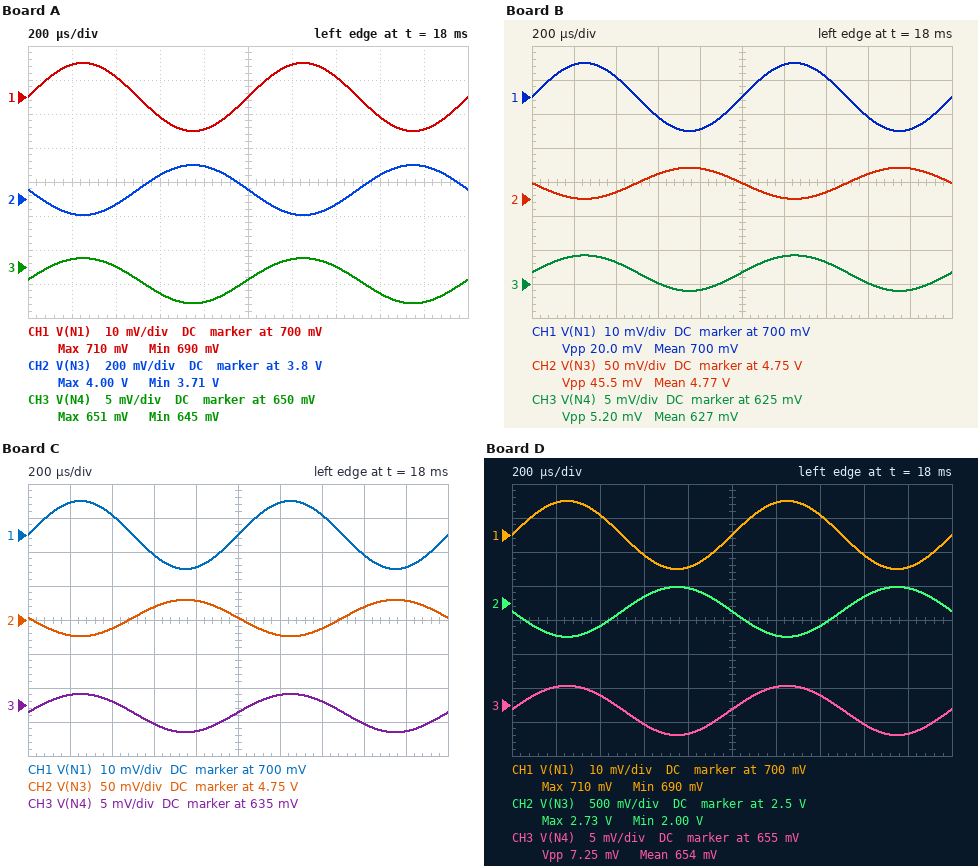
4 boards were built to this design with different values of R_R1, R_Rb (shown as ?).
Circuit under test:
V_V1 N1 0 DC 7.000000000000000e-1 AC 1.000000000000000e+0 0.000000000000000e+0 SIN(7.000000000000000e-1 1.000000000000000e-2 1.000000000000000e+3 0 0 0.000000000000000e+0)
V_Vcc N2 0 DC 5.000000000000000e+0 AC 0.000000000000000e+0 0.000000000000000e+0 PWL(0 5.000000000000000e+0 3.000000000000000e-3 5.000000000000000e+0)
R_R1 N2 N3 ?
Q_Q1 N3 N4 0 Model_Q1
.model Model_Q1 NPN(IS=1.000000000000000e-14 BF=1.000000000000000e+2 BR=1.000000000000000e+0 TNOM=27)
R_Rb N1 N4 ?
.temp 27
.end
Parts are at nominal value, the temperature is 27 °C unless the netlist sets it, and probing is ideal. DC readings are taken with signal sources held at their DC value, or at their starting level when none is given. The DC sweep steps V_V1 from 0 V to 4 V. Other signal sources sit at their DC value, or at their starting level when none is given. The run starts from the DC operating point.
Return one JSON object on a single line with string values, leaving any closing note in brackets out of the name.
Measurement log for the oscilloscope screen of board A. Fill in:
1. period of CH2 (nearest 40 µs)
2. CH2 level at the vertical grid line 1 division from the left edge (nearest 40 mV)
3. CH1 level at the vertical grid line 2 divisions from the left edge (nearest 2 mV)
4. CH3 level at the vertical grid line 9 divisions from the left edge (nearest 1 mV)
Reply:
{"period of CH2": "1.00 ms", "CH2 level at the vertical grid line 1 division from the left edge": "3.72 V", "CH1 level at the vertical grid line 2 divisions from the left edge": "706 mV", "CH3 level at the vertical grid line 9 divisions from the left edge": "645 mV"}
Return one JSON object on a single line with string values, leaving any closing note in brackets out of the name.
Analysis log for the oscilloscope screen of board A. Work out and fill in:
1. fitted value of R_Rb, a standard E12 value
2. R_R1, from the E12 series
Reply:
{"fitted value of R_Rb, a standard E12 value": "6.8 kΩ", "R_R1, from the E12 series": "1.5 kΩ"}
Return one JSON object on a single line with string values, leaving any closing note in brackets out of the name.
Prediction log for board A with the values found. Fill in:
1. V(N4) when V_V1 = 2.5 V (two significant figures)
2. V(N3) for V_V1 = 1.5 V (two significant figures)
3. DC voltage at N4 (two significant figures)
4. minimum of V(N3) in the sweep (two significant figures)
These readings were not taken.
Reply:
{"V(N4) when V_V1 = 2.5 V": "690 mV", "V(N3) for V_V1 = 1.5 V": "96 mV", "DC voltage at N4": "650 mV", "minimum of V(N3) in the sweep": "58 mV"}
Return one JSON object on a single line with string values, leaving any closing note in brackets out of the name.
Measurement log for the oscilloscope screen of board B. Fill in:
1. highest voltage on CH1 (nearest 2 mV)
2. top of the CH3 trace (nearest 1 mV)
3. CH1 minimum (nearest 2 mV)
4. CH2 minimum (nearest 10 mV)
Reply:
{"highest voltage on CH1": "710 mV", "top of the CH3 trace": "629 mV", "CH1 minimum": "690 mV", "CH2 minimum": "4.75 V"}
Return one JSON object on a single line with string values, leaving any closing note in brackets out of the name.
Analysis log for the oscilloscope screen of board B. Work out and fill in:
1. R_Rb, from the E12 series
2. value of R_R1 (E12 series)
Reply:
{"R_Rb, from the E12 series": "22 kΩ", "value of R_R1": "680 Ω"}
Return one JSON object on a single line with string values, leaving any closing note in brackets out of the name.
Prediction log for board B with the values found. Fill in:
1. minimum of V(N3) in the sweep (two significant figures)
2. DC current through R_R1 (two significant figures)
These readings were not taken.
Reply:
{"minimum of V(N3) in the sweep": "120 mV", "DC current through R_R1": "330 µA"}
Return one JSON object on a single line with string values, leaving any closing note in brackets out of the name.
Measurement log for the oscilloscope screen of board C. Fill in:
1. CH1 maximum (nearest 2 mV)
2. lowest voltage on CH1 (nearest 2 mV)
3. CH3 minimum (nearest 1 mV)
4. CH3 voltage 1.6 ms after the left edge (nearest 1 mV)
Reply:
{"CH1 maximum": "710 mV", "lowest voltage on CH1": "690 mV", "CH3 minimum": "631 mV", "CH3 voltage 1.6 ms after the left edge": "632 mV"}
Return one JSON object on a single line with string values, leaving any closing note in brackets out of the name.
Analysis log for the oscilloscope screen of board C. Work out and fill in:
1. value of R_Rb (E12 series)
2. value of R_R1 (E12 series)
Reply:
{"value of R_Rb": "15 kΩ", "value of R_R1": "560 Ω"}
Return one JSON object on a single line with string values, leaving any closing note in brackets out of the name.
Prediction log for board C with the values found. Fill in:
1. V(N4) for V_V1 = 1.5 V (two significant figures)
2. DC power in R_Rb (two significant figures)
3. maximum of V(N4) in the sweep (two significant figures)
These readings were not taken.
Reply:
{"V(N4) for V_V1 = 1.5 V": "700 mV", "DC power in R_Rb": "290 nW", "maximum of V(N4) in the sweep": "710 mV"}
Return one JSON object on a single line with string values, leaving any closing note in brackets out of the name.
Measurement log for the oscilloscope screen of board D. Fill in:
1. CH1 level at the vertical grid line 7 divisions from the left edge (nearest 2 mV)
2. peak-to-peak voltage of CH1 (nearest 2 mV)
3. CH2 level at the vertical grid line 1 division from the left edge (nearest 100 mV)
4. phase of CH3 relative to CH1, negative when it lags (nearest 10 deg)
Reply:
{"CH1 level at the vertical grid line 7 divisions from the left edge": "706 mV", "peak-to-peak voltage of CH1": "20 mV", "CH2 level at the vertical grid line 1 division from the left edge": "2.0 V", "phase of CH3 relative to CH1, negative when it lags": "0 deg"}
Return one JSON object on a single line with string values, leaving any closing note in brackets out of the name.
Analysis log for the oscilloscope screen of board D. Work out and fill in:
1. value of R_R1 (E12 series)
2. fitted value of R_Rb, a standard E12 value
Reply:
{"value of R_R1": "2.7 kΩ", "fitted value of R_Rb, a standard E12 value": "4.7 kΩ"}
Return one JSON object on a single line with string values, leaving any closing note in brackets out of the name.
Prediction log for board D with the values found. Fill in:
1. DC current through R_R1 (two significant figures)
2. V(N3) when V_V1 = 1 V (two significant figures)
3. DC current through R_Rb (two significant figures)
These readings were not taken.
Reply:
{"DC current through R_R1": "970 µA", "V(N3) when V_V1 = 1 V": "94 mV", "DC current through R_Rb": "9.7 µA"}
